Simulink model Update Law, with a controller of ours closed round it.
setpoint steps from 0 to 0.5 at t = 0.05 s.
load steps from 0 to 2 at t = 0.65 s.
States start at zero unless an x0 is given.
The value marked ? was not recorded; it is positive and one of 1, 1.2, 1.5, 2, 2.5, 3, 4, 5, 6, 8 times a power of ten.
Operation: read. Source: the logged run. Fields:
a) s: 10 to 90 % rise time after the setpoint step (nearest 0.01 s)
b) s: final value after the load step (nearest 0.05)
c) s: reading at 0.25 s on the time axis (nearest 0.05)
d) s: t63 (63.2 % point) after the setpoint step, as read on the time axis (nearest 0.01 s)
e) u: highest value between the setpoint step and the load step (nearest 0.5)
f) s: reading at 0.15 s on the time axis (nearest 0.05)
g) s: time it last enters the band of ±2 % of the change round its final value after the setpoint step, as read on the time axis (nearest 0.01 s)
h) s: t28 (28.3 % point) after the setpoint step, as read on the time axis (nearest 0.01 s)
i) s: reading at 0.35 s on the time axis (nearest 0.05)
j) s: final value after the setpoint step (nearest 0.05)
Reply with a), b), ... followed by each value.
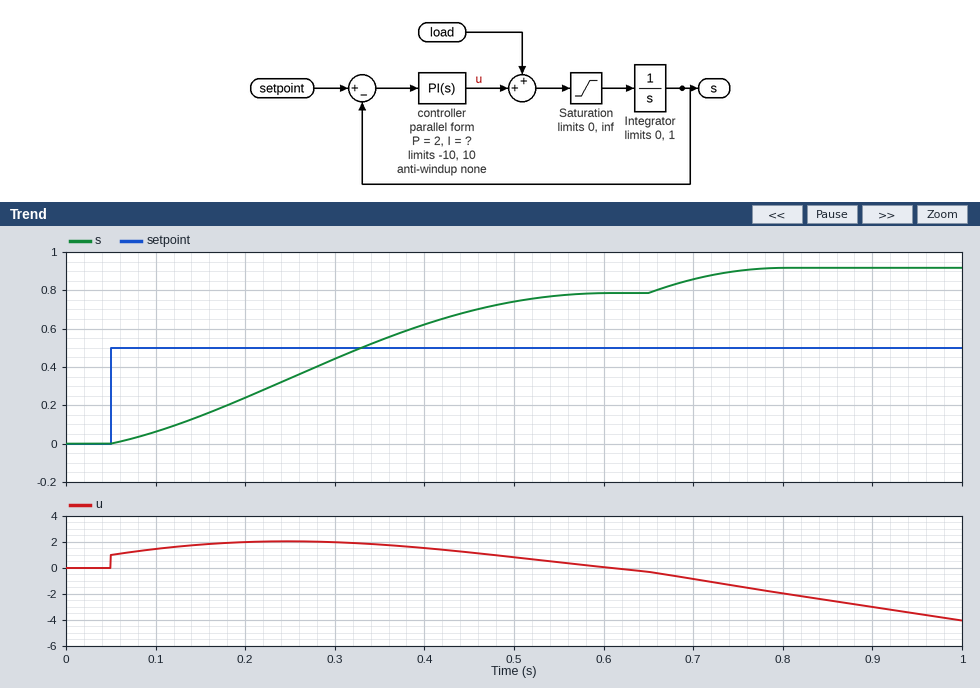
a) 0.35 s
b) 0.90
c) 0.35
d) 0.33 s
e) 2.0
f) 0.15
g) 0.54 s
h) 0.19 s
i) 0.55
j) 0.80
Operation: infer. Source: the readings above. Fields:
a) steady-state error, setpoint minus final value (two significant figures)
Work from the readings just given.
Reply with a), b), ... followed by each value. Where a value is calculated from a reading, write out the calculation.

a) 0.5 - 0.8 = -0.30
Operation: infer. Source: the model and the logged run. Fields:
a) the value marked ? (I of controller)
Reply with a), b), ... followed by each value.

a) 25
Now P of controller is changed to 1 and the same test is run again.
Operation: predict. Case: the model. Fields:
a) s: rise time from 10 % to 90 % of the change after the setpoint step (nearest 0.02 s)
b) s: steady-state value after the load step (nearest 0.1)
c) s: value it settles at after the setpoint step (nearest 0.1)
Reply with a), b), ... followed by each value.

a) 0.36 s
b) 1.0
c) 0.9
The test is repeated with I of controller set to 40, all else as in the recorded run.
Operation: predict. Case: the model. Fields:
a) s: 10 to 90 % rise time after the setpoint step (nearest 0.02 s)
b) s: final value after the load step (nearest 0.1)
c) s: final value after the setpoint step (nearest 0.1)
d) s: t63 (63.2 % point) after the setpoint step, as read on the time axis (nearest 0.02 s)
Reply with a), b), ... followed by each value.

a) 0.28 s
b) 0.8
c) 0.8
d) 0.28 s
